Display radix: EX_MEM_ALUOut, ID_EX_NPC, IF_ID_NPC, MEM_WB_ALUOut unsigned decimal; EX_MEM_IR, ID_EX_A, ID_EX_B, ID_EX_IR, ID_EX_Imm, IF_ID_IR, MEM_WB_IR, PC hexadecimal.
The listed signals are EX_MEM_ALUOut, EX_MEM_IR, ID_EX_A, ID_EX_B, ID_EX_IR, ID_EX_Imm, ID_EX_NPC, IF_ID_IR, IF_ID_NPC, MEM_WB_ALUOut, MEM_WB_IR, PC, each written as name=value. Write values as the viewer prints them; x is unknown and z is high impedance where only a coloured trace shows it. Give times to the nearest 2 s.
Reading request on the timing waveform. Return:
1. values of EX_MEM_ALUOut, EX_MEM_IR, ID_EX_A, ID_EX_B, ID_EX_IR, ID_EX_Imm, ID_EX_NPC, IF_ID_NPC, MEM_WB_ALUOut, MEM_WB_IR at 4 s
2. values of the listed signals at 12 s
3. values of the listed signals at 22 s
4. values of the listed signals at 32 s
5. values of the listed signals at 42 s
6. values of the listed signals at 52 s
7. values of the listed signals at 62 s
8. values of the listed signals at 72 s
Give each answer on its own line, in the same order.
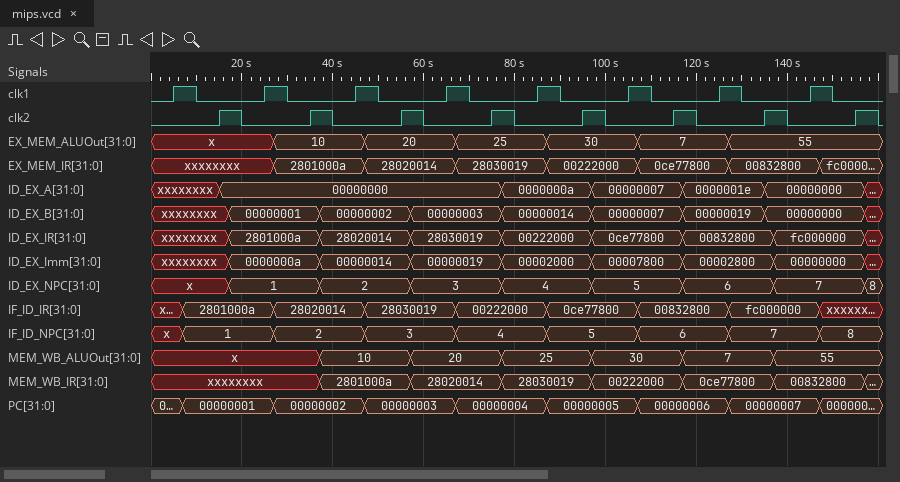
EX_MEM_ALUOut=x, EX_MEM_IR=xxxxxxxx, ID_EX_A=xxxxxxxx, ID_EX_B=xxxxxxxx, ID_EX_IR=xxxxxxxx, ID_EX_Imm=xxxxxxxx, ID_EX_NPC=x, IF_ID_NPC=x, MEM_WB_ALUOut=x, MEM_WB_IR=xxxxxxxx
EX_MEM_ALUOut=x, EX_MEM_IR=xxxxxxxx, ID_EX_A=xxxxxxxx, ID_EX_B=xxxxxxxx, ID_EX_IR=xxxxxxxx, ID_EX_Imm=xxxxxxxx, ID_EX_NPC=x, IF_ID_IR=2801000a, IF_ID_NPC=1, MEM_WB_ALUOut=x, MEM_WB_IR=xxxxxxxx, PC=00000001
EX_MEM_ALUOut=x, EX_MEM_IR=xxxxxxxx, ID_EX_A=00000000, ID_EX_B=00000001, ID_EX_IR=2801000a, ID_EX_Imm=0000000a, ID_EX_NPC=1, IF_ID_IR=2801000a, IF_ID_NPC=1, MEM_WB_ALUOut=x, MEM_WB_IR=xxxxxxxx, PC=00000001
EX_MEM_ALUOut=10, EX_MEM_IR=2801000a, ID_EX_A=00000000, ID_EX_B=00000001, ID_EX_IR=2801000a, ID_EX_Imm=0000000a, ID_EX_NPC=1, IF_ID_IR=28020014, IF_ID_NPC=2, MEM_WB_ALUOut=x, MEM_WB_IR=xxxxxxxx, PC=00000002
EX_MEM_ALUOut=10, EX_MEM_IR=2801000a, ID_EX_A=00000000, ID_EX_B=00000002, ID_EX_IR=28020014, ID_EX_Imm=00000014, ID_EX_NPC=2, IF_ID_IR=28020014, IF_ID_NPC=2, MEM_WB_ALUOut=10, MEM_WB_IR=2801000a, PC=00000002
EX_MEM_ALUOut=20, EX_MEM_IR=28020014, ID_EX_A=00000000, ID_EX_B=00000002, ID_EX_IR=28020014, ID_EX_Imm=00000014, ID_EX_NPC=2, IF_ID_IR=28030019, IF_ID_NPC=3, MEM_WB_ALUOut=10, MEM_WB_IR=2801000a, PC=00000003
EX_MEM_ALUOut=20, EX_MEM_IR=28020014, ID_EX_A=00000000, ID_EX_B=00000003, ID_EX_IR=28030019, ID_EX_Imm=00000019, ID_EX_NPC=3, IF_ID_IR=28030019, IF_ID_NPC=3, MEM_WB_ALUOut=20, MEM_WB_IR=28020014, PC=00000003
EX_MEM_ALUOut=25, EX_MEM_IR=28030019, ID_EX_A=00000000, ID_EX_B=00000003, ID_EX_IR=28030019, ID_EX_Imm=00000019, ID_EX_NPC=3, IF_ID_IR=00222000, IF_ID_NPC=4, MEM_WB_ALUOut=20, MEM_WB_IR=28020014, PC=00000004
